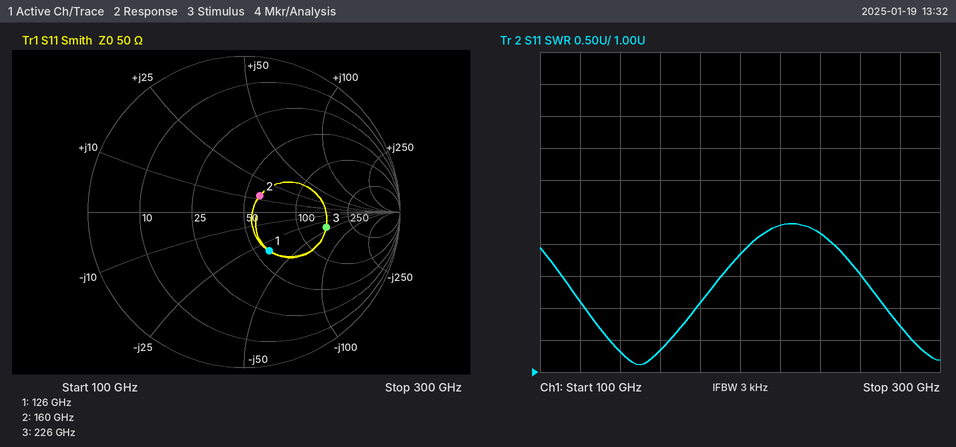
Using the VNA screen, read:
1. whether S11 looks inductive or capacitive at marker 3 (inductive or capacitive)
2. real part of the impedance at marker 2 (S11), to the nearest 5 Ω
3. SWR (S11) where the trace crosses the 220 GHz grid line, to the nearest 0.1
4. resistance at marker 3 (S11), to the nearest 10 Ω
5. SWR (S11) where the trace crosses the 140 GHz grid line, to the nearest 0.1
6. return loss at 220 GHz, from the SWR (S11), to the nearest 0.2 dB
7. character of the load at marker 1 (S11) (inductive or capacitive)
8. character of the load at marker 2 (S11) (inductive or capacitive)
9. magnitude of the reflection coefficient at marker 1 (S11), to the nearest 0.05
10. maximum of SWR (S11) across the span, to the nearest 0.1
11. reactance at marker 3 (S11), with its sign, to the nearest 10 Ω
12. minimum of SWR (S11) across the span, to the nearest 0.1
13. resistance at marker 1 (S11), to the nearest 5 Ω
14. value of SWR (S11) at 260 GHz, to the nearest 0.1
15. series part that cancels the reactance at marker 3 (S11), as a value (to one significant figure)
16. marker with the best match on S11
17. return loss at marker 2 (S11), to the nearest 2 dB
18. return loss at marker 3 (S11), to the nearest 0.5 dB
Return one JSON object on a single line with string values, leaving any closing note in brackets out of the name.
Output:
{"whether S11 looks inductive or capacitive at marker 3": "capacitive", "real part of the impedance at marker 2 (S11), to the nearest 5 Ω": "60 Ω", "SWR (S11) where the trace crosses the 220 GHz grid line, to the nearest 0.1": "3.3", "resistance at marker 3 (S11), to the nearest 10 Ω": "150 Ω", "SWR (S11) where the trace crosses the 140 GHz grid line, to the nearest 0.1": "1.3", "return loss at 220 GHz, from the SWR (S11), to the nearest 0.2 dB": "5.4 dB", "character of the load at marker 1 (S11)": "capacitive", "character of the load at marker 2 (S11)": "inductive", "magnitude of the reflection coefficient at marker 1 (S11), to the nearest 0.05": "0.30", "maximum of SWR (S11) across the span, to the nearest 0.1": "3.3", "reactance at marker 3 (S11), with its sign, to the nearest 10 Ω": "-40 Ω", "minimum of SWR (S11) across the span, to the nearest 0.1": "1.1", "resistance at marker 1 (S11), to the nearest 5 Ω": "60 Ω", "value of SWR (S11) at 260 GHz, to the nearest 0.1": "2.5", "series part that cancels the reactance at marker 3 (S11), as a value": "30 pH", "marker with the best match on S11": "marker 2", "return loss at marker 2 (S11), to the nearest 2 dB": "16 dB", "return loss at marker 3 (S11), to the nearest 0.5 dB": "5.5 dB"}
